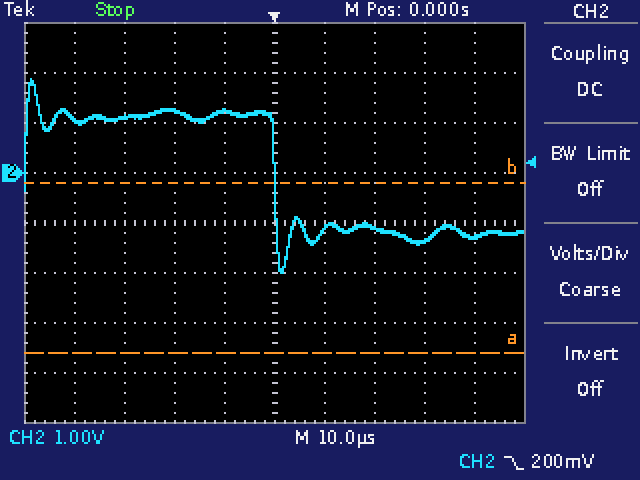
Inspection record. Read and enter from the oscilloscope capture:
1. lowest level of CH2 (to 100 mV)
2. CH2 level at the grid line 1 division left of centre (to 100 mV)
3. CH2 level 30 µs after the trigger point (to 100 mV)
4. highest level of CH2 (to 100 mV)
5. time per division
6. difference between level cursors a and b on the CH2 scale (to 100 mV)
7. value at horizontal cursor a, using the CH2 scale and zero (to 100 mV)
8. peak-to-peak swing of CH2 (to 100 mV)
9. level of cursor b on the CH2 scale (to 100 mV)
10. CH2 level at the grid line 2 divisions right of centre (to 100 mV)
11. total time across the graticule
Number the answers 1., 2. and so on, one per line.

1. -2.0 V
2. 1.2 V
3. -1.4 V
4. 1.9 V
5. 10 µs
6. 3.4 V
7. -3.6 V
8. 3.9 V
9. -200 mV
10. -1.1 V
11. 100 µs
